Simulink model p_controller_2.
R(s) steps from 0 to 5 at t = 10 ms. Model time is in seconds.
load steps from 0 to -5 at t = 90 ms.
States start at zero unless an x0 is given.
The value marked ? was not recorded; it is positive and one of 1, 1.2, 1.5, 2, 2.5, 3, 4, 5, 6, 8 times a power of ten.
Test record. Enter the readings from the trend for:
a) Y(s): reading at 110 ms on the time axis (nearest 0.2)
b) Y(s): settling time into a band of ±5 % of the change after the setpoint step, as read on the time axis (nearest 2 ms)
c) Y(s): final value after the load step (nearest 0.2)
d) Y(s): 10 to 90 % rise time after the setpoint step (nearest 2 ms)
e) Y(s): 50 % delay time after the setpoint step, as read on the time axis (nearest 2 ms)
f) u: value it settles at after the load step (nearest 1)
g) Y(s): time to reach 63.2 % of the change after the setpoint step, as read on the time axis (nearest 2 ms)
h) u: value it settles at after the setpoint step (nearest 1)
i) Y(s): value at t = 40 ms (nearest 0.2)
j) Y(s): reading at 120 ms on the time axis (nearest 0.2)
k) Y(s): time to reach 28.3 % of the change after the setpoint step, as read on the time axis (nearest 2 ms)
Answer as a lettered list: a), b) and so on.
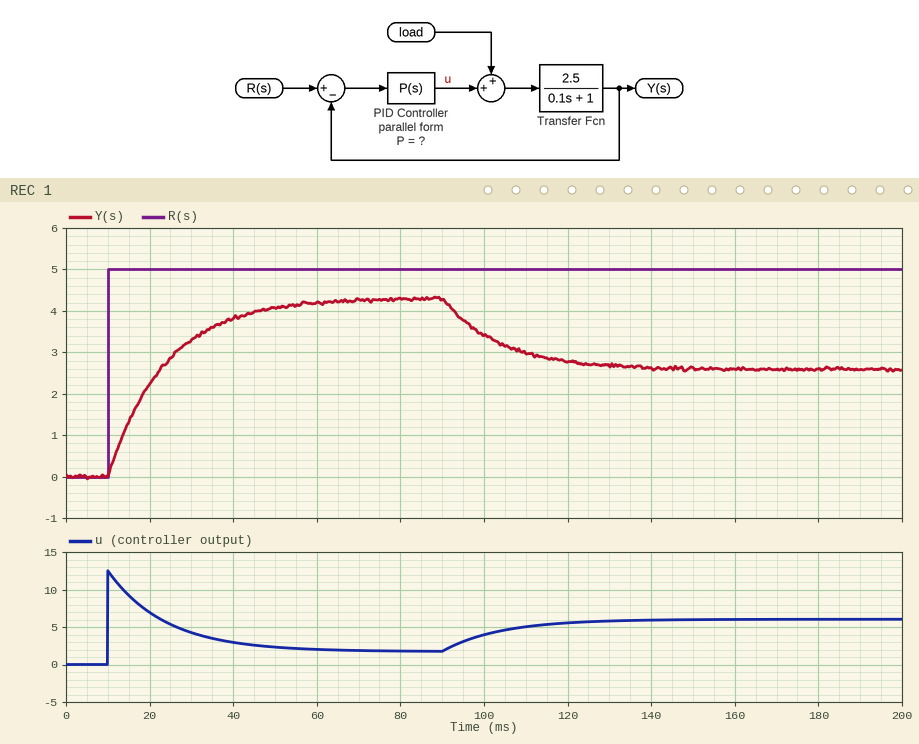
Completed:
a) 3.0
b) 52 ms
c) 2.6
d) 30 ms
e) 20 ms
f) 6
g) 24 ms
h) 2
i) 3.8
j) 2.8
k) 14 ms
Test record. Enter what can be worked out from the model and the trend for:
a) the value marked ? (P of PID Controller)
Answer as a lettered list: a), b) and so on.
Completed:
a) 2.5
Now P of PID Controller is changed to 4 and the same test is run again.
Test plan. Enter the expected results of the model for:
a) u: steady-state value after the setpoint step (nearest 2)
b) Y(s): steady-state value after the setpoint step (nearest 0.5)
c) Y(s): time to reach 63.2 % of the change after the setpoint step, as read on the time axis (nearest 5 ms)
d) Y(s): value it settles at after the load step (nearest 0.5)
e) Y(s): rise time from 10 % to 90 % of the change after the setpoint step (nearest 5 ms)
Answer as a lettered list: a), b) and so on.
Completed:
a) 2
b) 4.5
c) 20 ms
d) 3.5
e) 20 ms
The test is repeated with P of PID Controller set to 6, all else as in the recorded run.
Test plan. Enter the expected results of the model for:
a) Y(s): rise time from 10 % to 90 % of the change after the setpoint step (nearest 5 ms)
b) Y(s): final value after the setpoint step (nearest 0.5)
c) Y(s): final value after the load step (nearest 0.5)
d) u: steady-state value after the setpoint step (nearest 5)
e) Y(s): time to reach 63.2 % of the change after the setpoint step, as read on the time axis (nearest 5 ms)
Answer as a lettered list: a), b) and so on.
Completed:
a) 15 ms
b) 4.5
c) 4.0
d) 0
e) 15 ms
